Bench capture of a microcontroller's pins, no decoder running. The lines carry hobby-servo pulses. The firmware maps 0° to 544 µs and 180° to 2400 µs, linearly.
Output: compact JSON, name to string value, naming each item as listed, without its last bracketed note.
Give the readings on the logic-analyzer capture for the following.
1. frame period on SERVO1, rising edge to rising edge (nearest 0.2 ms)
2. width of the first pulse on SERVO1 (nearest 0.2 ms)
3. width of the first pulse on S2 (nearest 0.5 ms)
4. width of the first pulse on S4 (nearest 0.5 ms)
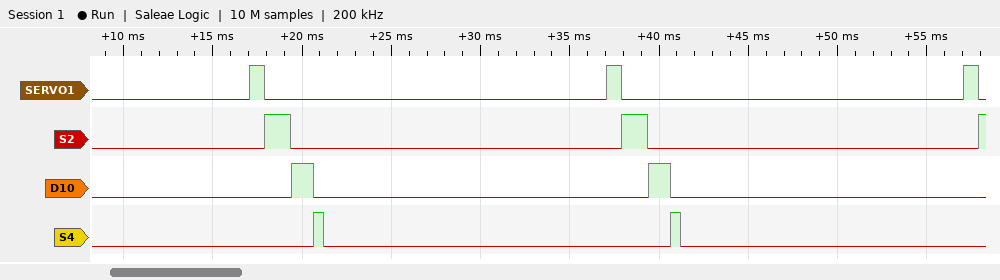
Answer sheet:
{"frame period on SERVO1, rising edge to rising edge": "20.0 ms", "width of the first pulse on SERVO1": "0.8 ms", "width of the first pulse on S2": "1.5 ms", "width of the first pulse on S4": "0.5 ms"}
